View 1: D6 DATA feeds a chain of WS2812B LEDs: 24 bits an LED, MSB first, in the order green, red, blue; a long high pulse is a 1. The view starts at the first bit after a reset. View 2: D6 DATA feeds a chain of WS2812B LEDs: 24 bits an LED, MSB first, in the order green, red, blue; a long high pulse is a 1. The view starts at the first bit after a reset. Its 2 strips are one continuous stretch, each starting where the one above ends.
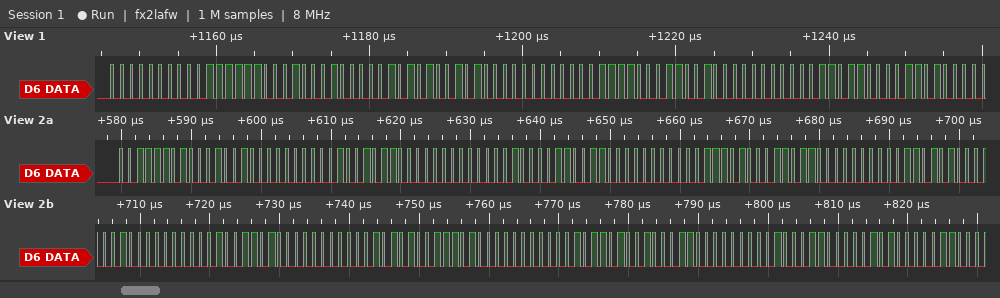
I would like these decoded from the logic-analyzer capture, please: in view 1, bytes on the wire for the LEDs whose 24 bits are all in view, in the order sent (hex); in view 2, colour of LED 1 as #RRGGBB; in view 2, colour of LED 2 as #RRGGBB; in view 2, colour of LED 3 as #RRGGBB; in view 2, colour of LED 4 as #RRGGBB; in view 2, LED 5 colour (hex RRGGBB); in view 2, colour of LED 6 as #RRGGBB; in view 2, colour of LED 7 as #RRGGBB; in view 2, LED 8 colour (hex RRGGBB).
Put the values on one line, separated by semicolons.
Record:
00 3F 11 05 4A 00 1E 32 00; #123D00; #004B04; #00331D; #001B35; #00024D; #15003A; #2D0023; #46000A
